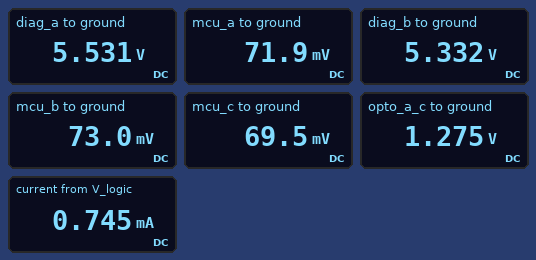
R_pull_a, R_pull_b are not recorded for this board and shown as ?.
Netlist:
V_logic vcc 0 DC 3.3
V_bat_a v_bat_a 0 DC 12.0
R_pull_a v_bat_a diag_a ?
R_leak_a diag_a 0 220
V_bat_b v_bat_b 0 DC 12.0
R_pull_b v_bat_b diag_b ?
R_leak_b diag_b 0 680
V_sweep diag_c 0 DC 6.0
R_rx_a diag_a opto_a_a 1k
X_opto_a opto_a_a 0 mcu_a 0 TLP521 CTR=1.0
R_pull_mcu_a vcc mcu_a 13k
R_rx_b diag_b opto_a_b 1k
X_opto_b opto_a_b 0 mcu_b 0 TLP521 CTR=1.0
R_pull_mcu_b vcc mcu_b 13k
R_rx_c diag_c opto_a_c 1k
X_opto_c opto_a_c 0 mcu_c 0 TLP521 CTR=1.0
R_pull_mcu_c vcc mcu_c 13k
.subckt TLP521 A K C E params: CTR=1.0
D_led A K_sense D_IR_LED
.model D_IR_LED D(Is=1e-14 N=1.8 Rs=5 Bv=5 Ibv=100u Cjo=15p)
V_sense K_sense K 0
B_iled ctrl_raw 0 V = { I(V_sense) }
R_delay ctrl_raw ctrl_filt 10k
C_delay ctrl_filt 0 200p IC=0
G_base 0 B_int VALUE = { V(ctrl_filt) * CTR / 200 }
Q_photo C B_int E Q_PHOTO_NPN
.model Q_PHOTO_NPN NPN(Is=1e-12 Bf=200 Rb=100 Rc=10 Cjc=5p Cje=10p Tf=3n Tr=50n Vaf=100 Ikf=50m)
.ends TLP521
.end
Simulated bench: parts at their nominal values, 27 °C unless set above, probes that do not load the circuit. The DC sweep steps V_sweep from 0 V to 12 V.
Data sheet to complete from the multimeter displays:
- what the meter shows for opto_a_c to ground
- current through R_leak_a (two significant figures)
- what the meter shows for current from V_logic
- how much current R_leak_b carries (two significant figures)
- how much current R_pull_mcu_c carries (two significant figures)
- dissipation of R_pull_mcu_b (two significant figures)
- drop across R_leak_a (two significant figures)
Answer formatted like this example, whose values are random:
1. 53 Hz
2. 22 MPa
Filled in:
1. 1.275 V
2. 25 mA
3. 0.745 mA
4. 7.8 mA
5. 250 µA
6. 800 µW
7. 5.5 V
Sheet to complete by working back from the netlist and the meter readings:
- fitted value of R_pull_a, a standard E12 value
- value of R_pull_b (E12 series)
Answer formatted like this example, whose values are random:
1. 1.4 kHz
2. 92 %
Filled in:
1. 220 Ω
2. 560 Ω
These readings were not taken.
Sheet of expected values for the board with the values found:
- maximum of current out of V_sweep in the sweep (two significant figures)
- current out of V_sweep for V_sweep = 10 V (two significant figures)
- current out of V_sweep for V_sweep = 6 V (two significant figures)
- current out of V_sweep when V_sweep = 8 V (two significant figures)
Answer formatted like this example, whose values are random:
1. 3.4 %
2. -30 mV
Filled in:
1. 11 mA
2. 8.7 mA
3. 4.7 mA
4. 6.7 mA
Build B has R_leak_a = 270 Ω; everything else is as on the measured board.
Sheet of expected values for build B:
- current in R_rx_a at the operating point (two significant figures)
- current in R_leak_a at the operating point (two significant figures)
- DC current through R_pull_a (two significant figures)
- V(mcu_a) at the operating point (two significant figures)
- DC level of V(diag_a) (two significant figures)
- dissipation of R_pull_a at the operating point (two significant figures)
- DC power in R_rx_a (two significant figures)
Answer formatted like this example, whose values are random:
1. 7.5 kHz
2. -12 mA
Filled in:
1. 4.8 mA
2. 22 mA
3. 27 mA
4. 69 mV
5. 6.0 V
6. 160 mW
7. 23 mW
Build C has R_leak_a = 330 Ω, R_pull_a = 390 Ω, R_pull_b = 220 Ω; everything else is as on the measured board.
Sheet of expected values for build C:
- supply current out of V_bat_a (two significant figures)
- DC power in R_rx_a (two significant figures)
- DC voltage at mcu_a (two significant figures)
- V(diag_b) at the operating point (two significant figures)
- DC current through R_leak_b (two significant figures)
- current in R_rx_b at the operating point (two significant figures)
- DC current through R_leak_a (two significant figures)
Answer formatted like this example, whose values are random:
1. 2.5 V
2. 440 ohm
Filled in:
1. 18 mA
2. 13 mW
3. 76 mV
4. 8.0 V
5. 12 mA
6. 6.7 mA
7. 15 mA
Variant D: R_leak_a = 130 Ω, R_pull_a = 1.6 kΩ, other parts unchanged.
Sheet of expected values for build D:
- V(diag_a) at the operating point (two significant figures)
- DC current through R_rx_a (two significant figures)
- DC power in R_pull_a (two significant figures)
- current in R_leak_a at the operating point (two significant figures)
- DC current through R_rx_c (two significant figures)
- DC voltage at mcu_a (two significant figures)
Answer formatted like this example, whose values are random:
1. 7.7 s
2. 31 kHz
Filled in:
1. 900 mV
2. 2.4 µA
3. 77 mW
4. 6.9 mA
5. 4.7 mA
6. 3.3 V
